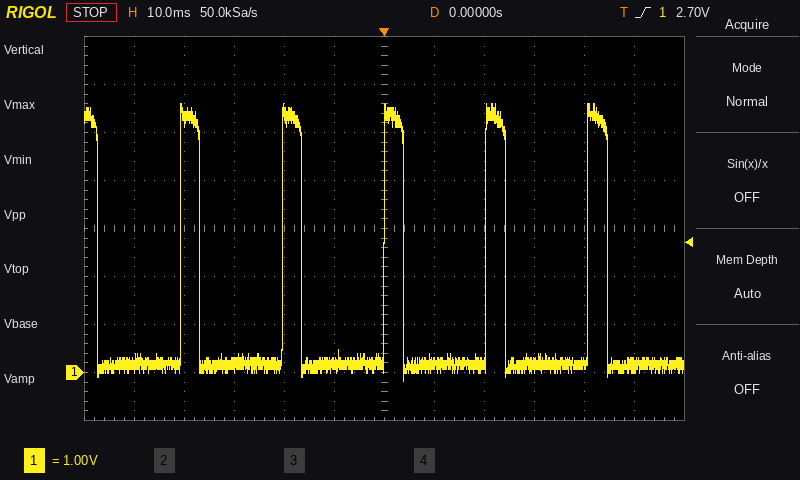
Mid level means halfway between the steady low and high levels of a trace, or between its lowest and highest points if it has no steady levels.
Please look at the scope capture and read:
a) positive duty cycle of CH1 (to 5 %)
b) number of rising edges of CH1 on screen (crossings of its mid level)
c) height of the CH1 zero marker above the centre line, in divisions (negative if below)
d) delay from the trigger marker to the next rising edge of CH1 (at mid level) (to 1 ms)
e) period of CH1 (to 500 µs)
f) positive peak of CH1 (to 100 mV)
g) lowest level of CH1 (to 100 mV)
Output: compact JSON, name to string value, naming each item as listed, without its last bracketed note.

{"positive duty cycle of CH1": "20 %", "number of rising edges of CH1 on screen": "5", "height of the CH1 zero marker above the centre line, in divisions": "-3.0 div", "delay from the trigger marker to the next rising edge of CH1 (at mid level)": "20 ms", "period of CH1": "20.5 ms", "positive peak of CH1": "5.6 V", "lowest level of CH1": "-200 mV"}
